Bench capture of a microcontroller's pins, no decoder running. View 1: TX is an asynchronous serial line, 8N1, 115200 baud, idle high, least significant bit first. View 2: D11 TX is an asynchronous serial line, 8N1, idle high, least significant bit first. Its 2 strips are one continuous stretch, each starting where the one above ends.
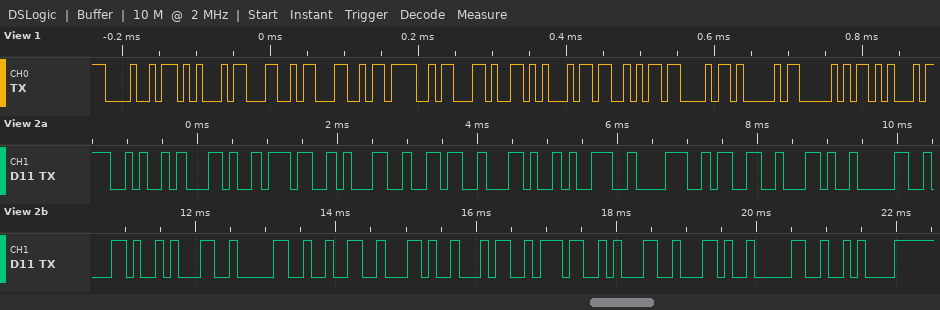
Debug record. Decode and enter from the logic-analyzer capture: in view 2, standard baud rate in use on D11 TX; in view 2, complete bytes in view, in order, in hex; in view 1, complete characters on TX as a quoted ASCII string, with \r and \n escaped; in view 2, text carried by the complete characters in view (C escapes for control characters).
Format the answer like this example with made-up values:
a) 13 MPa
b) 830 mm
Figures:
a) 9600 baud
b) 4A 2C 37 31 36 2C 39 38 33 2C 30 2C 31 30 32 2C 34 37 31 2C 30 0A
c) "HELLO,ESCAPE"
d) "J,716,983,0,102,471,0\n"
